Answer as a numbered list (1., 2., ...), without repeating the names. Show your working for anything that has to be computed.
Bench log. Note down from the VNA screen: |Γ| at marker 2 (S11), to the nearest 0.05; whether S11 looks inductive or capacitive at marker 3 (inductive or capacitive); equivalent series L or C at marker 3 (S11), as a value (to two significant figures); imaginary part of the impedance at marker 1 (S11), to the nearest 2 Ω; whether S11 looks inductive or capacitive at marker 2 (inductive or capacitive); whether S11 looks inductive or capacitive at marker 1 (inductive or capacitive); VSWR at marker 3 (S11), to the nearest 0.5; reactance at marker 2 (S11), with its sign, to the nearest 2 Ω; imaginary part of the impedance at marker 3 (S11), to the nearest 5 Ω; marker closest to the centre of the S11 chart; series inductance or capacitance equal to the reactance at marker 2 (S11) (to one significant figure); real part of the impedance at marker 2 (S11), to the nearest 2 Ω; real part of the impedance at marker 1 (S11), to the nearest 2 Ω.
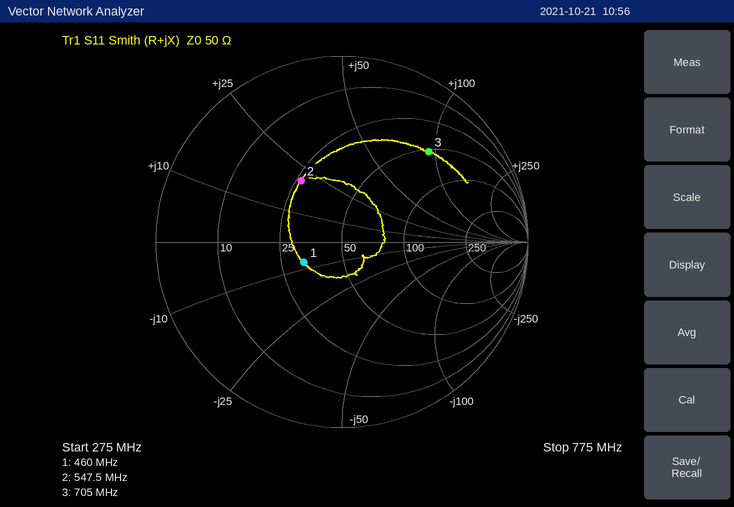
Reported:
1. 0.40
2. inductive
3. L = 95 Ω/(2π × 705 MHz) ≈ 21 nH
4. -8 Ω
5. inductive
6. capacitive
7. 5.0
8. +20 Ω
9. +95 Ω
10. marker 1
11. L = 20 Ω/(2π × 547.5 MHz) ≈ 6 nH
12. 26 Ω
13. 32 Ω
